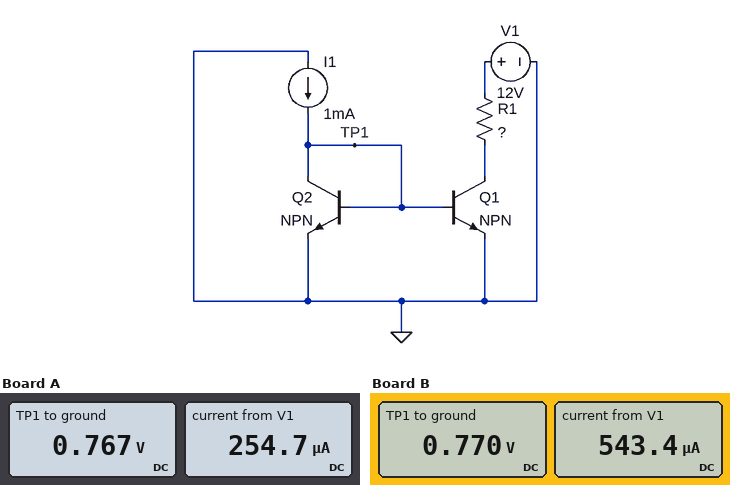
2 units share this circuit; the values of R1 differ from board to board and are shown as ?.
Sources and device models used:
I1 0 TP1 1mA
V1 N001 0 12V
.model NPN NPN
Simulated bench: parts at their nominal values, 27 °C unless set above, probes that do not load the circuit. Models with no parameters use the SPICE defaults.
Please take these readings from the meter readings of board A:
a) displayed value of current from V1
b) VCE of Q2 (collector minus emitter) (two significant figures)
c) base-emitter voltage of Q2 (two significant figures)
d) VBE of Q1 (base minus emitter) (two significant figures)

254.7 µA
770 mV
770 mV
770 mV
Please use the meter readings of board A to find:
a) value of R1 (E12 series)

47 kΩ
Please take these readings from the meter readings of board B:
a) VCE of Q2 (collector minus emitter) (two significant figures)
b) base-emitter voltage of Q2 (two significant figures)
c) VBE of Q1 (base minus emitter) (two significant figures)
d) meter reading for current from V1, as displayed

770 mV
770 mV
770 mV
543.4 µA
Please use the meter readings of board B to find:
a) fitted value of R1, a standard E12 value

22 kΩ
